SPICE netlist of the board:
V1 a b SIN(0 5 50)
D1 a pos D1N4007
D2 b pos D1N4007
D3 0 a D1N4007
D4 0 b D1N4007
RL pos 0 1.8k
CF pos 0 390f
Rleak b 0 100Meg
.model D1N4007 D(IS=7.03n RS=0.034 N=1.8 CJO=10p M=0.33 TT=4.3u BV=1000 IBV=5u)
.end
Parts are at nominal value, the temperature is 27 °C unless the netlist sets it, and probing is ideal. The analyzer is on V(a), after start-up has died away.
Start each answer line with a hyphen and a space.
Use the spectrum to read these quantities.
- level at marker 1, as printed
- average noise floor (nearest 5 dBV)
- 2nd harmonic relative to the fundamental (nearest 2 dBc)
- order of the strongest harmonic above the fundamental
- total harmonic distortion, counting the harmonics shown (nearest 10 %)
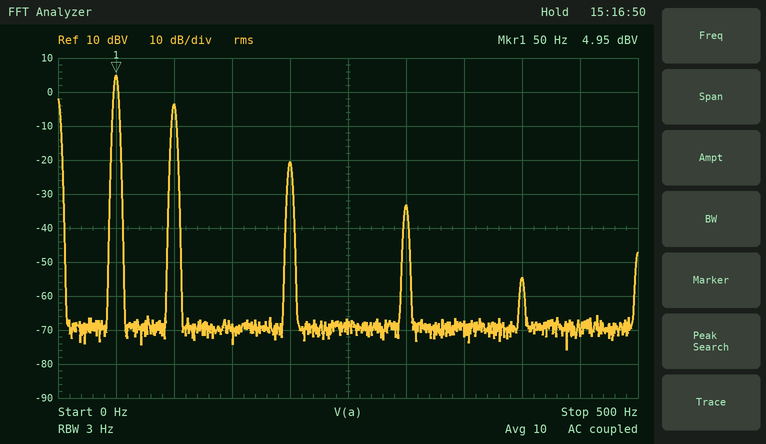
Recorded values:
- 4.95 dBV
- -70 dBV
- -8 dBc
- 2
- 40 %
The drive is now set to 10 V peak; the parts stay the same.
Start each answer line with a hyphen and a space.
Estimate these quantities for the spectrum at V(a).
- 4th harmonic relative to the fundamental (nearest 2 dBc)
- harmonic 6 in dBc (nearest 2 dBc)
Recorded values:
- -22 dBc
- -32 dBc
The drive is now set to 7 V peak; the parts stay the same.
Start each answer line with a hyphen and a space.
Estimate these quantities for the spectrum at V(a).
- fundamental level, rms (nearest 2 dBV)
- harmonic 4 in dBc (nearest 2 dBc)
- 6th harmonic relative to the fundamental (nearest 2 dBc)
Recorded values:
- 8 dBV
- -24 dBc
- -34 dBc
